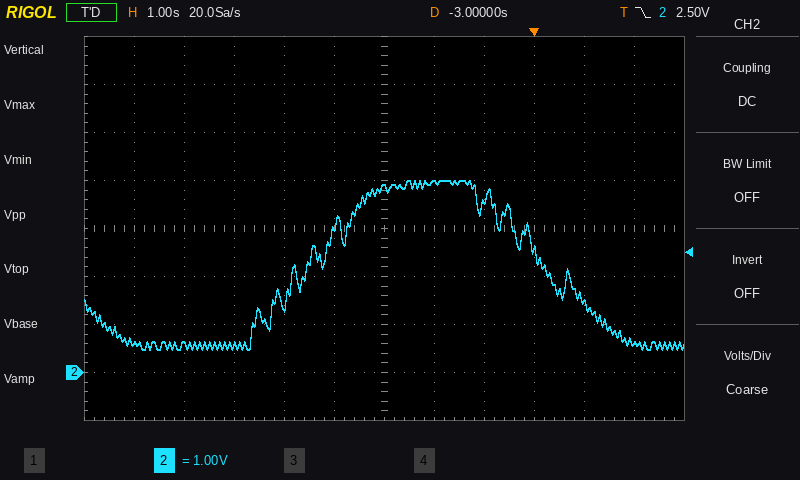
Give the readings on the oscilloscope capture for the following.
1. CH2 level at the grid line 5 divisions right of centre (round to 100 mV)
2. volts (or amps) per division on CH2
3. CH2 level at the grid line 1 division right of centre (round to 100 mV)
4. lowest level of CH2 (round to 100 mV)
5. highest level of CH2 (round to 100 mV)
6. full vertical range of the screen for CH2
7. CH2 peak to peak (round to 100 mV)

600 mV
1 V
4.0 V
500 mV
4.0 V
8 V
3.5 V
